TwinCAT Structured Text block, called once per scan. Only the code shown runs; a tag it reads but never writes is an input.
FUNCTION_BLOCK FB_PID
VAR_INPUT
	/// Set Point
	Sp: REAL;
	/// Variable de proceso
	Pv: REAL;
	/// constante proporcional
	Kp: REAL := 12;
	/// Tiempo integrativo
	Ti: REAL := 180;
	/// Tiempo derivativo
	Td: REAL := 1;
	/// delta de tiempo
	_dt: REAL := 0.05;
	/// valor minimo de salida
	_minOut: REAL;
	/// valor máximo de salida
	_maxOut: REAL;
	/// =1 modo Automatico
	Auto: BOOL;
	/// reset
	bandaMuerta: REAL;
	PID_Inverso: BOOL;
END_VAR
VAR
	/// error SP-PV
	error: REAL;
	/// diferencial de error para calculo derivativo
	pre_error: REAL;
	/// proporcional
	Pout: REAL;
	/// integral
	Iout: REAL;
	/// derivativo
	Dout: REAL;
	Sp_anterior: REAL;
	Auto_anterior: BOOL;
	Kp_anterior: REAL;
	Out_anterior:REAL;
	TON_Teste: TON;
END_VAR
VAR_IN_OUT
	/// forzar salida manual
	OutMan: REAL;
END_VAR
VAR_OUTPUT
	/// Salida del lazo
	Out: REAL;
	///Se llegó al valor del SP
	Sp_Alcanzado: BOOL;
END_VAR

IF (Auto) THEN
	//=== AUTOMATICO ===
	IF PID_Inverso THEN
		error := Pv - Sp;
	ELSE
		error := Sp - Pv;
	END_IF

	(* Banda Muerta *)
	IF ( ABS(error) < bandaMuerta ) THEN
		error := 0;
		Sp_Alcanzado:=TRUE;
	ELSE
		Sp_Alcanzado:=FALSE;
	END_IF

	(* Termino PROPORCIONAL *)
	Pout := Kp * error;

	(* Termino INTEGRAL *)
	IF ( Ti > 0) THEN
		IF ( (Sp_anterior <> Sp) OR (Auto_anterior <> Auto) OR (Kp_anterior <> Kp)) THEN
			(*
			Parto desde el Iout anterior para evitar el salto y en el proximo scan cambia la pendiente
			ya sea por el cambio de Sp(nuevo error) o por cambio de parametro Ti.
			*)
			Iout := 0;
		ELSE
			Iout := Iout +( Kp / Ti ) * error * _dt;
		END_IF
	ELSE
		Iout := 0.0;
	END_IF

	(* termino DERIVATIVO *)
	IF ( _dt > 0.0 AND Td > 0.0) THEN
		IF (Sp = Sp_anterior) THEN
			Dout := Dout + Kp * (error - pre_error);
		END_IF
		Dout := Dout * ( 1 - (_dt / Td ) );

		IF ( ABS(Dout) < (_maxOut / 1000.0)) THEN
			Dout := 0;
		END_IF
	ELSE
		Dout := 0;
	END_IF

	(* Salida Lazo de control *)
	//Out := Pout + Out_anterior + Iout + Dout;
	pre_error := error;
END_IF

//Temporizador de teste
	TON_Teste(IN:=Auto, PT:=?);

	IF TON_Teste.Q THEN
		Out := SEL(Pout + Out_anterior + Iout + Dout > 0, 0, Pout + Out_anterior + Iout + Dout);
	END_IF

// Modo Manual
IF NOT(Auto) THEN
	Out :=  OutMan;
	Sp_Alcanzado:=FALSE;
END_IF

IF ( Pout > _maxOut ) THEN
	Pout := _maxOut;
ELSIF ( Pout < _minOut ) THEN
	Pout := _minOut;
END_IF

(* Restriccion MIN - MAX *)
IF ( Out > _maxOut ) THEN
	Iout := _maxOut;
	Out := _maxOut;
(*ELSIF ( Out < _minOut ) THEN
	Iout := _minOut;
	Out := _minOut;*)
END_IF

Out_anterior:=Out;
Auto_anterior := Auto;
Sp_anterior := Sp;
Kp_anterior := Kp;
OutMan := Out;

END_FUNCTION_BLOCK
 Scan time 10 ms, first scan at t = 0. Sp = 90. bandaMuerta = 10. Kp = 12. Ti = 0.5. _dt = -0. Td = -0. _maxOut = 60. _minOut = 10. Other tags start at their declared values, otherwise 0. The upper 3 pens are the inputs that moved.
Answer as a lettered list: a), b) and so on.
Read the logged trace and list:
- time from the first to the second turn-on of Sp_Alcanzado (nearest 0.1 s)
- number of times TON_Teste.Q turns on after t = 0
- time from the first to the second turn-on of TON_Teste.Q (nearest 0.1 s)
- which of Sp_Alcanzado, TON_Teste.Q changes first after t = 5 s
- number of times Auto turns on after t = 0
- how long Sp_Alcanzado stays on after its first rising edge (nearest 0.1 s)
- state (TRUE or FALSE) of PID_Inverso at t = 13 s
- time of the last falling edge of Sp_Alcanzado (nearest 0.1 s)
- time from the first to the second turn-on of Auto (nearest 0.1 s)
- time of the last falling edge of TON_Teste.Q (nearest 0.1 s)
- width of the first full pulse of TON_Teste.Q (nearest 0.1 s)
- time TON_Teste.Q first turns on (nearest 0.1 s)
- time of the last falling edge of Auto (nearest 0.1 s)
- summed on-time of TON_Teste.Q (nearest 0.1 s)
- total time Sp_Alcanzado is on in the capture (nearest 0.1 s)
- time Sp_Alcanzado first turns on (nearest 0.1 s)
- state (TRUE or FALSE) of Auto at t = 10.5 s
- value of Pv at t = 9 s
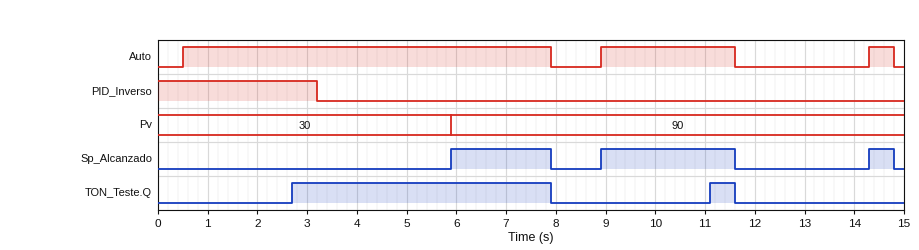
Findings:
a) 3.0 s
b) 2
c) 8.4 s
d) Sp_Alcanzado
e) 3
f) 2.0 s
g) FALSE
h) 14.8 s
i) 8.4 s
j) 11.6 s
k) 5.2 s
l) 2.7 s
m) 14.8 s
n) 5.7 s
o) 5.2 s
p) 5.9 s
q) TRUE
r) 90
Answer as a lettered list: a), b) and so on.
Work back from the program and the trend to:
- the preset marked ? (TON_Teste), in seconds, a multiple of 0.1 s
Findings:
a) 2.2 s
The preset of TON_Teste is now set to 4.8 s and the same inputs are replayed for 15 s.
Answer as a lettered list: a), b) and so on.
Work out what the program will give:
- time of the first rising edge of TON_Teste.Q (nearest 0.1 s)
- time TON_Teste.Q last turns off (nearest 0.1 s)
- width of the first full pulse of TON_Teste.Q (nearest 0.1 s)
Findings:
a) 5.3 s
b) 7.9 s
c) 2.6 s
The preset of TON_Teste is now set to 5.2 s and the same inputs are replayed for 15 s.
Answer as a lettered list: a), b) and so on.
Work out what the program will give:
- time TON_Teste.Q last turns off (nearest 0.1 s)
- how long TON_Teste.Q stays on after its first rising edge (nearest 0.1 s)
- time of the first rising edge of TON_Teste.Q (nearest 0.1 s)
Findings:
a) 7.9 s
b) 2.2 s
c) 5.7 s
